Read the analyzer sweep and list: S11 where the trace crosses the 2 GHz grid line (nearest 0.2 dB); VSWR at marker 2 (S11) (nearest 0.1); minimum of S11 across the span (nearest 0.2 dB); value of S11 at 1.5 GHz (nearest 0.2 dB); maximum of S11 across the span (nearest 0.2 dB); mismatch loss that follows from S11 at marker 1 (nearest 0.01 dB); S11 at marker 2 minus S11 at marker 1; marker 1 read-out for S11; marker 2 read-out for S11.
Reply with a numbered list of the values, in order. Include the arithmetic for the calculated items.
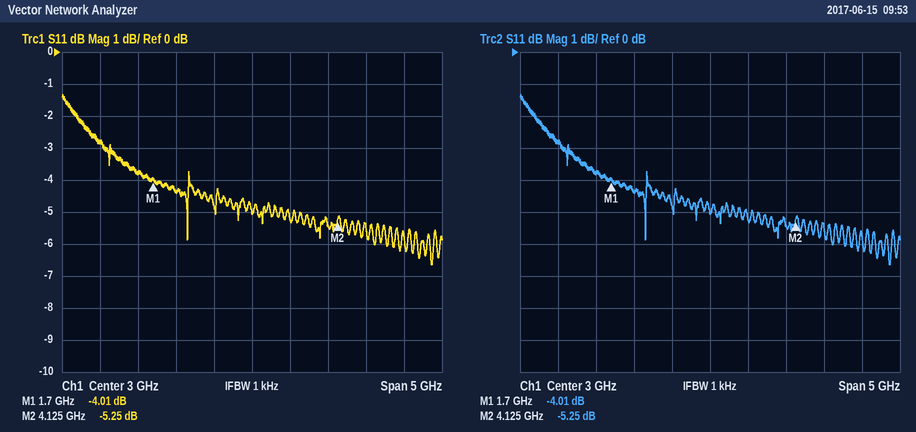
1. -4.4 dB
2. (1 + 0.5464)/(1 − 0.5464) ≈ 3.4
3. -6.6 dB
4. -3.8 dB
5. -1.4 dB
6. −10 log10(1 − 10^(-4.01/10)) ≈ 2.20 dB
7. -5.25 − (-4.01) = -1.24 dB
8. -4.01 dB
9. -5.25 dB
